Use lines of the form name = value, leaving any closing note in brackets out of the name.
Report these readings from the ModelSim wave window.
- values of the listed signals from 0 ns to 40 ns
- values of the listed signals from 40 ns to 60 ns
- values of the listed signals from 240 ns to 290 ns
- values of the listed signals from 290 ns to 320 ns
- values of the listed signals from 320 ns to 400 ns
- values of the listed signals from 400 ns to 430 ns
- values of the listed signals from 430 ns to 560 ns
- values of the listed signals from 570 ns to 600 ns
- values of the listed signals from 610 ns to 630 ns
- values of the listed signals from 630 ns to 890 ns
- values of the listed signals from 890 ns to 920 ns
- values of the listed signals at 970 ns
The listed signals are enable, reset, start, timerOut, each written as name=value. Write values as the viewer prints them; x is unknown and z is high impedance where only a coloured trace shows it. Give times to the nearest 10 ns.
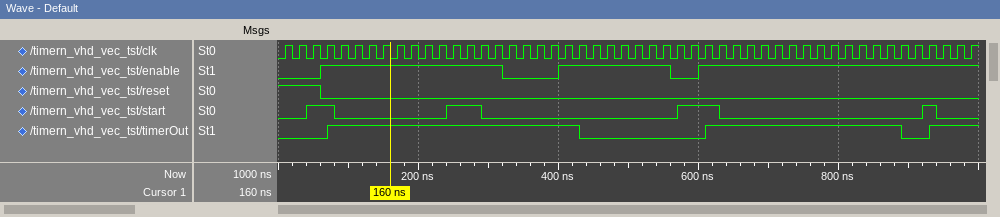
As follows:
values of the listed signals from 0 ns to 40 ns = enable=0, reset=1, start=0, timerOut=0
values of the listed signals from 40 ns to 60 ns = enable=0, reset=1, start=1, timerOut=0
values of the listed signals from 240 ns to 290 ns = enable=1, reset=0, start=1, timerOut=1
values of the listed signals from 290 ns to 320 ns = enable=1, reset=0, start=0, timerOut=1
values of the listed signals from 320 ns to 400 ns = enable=0, reset=0, start=0, timerOut=1
values of the listed signals from 400 ns to 430 ns = enable=1, reset=0, start=0, timerOut=1
values of the listed signals from 430 ns to 560 ns = enable=1, reset=0, start=0, timerOut=0
values of the listed signals from 570 ns to 600 ns = enable=0, reset=0, start=1, timerOut=0
values of the listed signals from 610 ns to 630 ns = enable=1, reset=0, start=1, timerOut=1
values of the listed signals from 630 ns to 890 ns = enable=1, reset=0, start=0, timerOut=1
values of the listed signals from 890 ns to 920 ns = enable=1, reset=0, start=0, timerOut=0
values of the listed signals at 970 ns = enable=1, reset=0, start=0, timerOut=1
